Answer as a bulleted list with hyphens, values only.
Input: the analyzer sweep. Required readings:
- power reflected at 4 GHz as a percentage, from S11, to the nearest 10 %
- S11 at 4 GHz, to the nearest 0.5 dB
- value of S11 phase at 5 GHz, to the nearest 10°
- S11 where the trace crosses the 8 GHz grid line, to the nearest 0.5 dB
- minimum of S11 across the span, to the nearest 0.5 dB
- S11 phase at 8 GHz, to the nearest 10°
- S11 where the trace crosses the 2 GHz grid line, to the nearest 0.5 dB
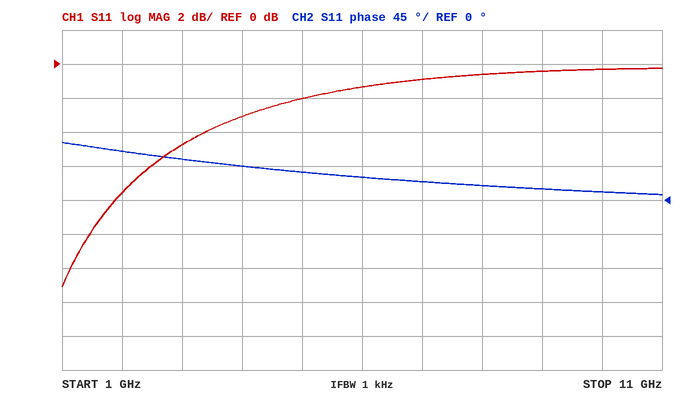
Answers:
- 50 %
- -3.0 dB
- 40°
- -0.5 dB
- -13.0 dB
- 20°
- -7.5 dB
